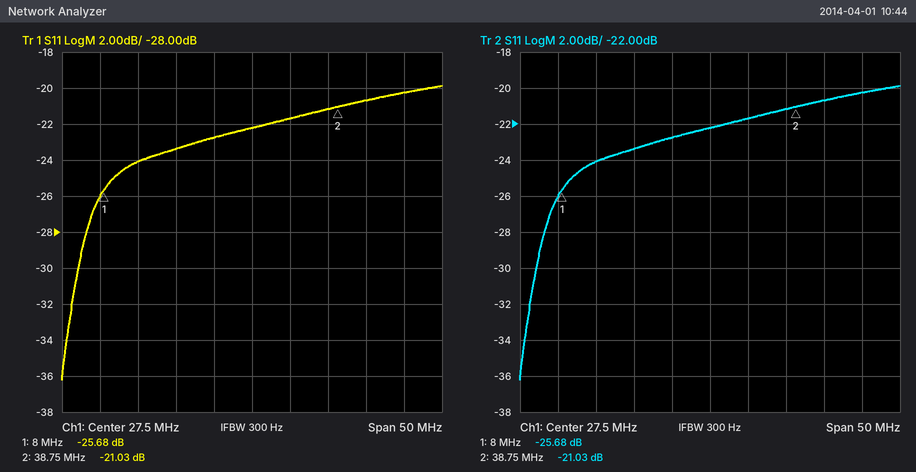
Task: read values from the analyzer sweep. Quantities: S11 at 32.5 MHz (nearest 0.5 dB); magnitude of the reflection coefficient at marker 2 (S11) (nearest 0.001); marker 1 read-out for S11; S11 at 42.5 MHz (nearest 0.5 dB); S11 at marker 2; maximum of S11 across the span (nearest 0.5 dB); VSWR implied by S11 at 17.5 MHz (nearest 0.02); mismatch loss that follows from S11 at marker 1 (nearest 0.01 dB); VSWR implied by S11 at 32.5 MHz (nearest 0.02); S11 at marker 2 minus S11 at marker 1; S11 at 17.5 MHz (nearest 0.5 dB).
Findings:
-21.5 dB
0.089
-25.68 dB
-20.5 dB
-21.03 dB
-20.0 dB
1.14
0.01 dB
1.18
4.65 dB
-23.5 dB
